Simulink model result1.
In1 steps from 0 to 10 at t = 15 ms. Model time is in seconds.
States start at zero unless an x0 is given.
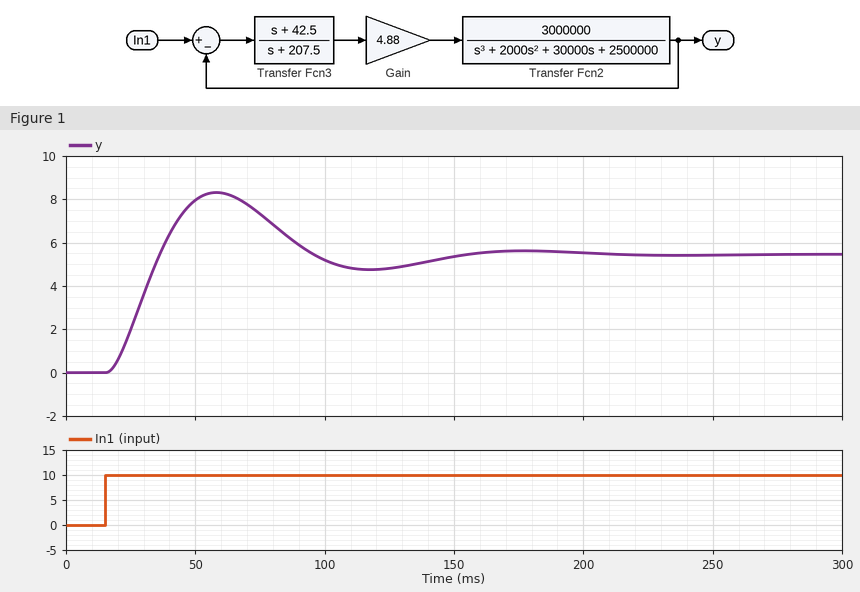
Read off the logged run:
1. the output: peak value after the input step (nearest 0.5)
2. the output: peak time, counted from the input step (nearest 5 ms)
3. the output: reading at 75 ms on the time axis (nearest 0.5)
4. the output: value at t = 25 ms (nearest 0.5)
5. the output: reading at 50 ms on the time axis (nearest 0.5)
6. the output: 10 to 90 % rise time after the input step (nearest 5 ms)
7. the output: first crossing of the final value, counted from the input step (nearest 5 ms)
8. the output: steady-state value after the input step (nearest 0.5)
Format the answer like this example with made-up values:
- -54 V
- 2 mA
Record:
- 8.5
- 45 ms
- 7.5
- 2.0
- 8.0
- 15 ms
- 20 ms
- 5.5
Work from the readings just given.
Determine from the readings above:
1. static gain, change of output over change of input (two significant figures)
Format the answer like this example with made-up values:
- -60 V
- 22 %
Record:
- 0.55
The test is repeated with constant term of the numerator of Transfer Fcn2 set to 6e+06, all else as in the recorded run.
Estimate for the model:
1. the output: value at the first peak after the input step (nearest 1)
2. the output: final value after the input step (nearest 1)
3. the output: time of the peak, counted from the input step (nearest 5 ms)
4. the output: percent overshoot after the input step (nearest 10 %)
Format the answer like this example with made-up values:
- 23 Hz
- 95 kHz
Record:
- 10
- 7
- 30 ms
- 50 %
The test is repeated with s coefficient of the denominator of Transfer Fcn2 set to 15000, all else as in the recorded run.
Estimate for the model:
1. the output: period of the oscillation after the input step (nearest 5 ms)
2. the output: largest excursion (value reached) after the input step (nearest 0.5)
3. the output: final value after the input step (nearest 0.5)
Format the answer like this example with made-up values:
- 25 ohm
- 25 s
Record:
- 115 ms
- 9.0
- 5.5
